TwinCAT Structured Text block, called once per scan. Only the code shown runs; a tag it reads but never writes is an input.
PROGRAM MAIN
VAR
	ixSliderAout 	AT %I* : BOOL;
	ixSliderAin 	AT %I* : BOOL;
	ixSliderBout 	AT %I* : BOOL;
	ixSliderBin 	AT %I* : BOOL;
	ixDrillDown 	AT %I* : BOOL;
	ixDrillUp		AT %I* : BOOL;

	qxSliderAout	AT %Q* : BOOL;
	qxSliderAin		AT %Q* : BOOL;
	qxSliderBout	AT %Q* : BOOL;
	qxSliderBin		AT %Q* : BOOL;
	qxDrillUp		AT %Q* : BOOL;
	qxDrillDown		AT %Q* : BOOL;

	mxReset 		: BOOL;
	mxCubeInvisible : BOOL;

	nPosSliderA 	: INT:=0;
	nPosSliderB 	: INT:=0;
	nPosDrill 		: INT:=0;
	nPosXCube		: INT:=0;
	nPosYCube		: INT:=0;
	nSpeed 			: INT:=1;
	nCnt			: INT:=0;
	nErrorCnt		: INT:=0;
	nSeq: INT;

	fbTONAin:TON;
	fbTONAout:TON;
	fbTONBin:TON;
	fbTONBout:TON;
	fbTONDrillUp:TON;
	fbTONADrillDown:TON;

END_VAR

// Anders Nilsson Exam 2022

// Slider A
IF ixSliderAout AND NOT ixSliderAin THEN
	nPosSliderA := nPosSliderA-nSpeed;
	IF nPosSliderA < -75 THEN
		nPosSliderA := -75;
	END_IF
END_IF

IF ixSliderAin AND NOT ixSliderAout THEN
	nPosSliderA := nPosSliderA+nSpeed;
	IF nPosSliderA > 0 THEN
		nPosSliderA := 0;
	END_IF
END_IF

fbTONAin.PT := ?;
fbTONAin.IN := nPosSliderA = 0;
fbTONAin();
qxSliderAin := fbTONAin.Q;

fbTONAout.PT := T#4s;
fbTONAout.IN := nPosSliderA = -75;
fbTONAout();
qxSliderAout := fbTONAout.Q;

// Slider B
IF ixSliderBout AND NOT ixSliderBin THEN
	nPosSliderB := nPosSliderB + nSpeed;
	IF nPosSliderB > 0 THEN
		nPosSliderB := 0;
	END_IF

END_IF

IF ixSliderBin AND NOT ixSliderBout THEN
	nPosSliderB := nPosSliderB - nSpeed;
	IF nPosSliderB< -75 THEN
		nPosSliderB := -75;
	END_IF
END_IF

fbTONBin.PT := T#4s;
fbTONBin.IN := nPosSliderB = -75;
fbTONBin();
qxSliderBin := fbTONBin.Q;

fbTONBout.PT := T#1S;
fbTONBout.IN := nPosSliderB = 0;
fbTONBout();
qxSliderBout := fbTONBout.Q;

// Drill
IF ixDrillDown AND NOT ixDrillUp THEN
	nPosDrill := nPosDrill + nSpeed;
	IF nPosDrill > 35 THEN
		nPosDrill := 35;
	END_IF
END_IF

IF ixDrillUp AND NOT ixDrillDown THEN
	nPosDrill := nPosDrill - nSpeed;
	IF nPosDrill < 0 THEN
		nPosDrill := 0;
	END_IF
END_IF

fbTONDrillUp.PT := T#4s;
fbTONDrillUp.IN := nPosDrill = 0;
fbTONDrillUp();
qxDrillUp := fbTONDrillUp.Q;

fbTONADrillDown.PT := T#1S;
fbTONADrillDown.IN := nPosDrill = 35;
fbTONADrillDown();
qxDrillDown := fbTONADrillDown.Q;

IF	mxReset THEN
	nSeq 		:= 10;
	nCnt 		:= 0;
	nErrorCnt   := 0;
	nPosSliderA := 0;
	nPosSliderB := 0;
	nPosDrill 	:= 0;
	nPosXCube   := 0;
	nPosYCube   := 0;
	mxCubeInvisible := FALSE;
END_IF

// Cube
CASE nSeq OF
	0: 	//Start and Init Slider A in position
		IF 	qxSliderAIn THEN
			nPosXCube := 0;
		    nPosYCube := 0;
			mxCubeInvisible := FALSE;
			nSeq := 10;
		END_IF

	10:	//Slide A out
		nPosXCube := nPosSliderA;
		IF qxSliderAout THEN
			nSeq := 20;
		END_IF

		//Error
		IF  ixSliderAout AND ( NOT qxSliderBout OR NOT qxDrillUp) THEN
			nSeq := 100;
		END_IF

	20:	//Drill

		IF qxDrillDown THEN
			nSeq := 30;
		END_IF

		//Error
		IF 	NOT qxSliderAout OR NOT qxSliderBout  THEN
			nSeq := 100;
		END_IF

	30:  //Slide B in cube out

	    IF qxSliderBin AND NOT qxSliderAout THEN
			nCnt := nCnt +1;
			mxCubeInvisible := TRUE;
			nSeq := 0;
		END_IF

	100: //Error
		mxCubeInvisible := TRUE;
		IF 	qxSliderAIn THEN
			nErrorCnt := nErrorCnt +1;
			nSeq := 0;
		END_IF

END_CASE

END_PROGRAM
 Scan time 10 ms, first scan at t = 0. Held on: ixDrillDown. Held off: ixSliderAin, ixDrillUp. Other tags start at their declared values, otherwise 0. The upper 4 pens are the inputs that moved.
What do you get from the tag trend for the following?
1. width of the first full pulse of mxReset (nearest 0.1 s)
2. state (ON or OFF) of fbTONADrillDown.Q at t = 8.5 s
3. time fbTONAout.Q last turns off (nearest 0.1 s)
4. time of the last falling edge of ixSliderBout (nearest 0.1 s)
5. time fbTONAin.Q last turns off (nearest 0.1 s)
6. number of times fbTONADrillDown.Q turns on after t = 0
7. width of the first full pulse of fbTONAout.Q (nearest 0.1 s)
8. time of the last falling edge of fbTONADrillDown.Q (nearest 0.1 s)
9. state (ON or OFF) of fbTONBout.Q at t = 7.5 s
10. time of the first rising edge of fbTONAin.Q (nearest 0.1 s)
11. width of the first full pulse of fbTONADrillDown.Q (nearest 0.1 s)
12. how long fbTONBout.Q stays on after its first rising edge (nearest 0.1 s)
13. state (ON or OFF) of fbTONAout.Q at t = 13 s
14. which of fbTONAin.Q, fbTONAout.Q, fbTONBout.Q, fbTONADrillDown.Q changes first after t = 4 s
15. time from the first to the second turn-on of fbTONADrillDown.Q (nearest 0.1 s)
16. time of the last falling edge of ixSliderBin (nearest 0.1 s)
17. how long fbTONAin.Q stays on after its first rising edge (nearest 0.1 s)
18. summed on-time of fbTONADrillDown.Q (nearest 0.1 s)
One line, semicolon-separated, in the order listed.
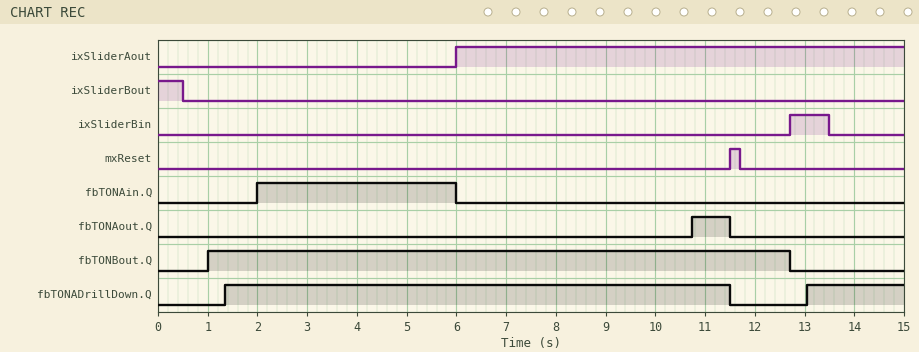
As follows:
0.2 s; ON; 11.5 s; 0.5 s; 6.0 s; 2; 0.8 s; 11.5 s; ON; 2.0 s; 10.2 s; 11.7 s; OFF; fbTONAin.Q; 11.7 s; 13.5 s; 4.0 s; 12.1 s
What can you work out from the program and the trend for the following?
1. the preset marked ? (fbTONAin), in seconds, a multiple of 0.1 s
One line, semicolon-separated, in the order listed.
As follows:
2.0 s
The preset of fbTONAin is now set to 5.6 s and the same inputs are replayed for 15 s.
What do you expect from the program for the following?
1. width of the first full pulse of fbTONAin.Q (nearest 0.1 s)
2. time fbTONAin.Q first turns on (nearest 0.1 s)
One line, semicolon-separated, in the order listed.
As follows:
0.4 s; 5.6 s
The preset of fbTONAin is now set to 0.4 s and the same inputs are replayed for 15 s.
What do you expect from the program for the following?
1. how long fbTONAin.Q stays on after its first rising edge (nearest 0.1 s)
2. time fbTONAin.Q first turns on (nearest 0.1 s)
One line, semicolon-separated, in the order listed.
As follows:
5.6 s; 0.4 s
